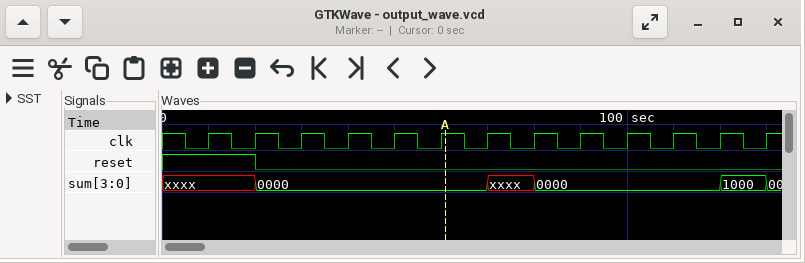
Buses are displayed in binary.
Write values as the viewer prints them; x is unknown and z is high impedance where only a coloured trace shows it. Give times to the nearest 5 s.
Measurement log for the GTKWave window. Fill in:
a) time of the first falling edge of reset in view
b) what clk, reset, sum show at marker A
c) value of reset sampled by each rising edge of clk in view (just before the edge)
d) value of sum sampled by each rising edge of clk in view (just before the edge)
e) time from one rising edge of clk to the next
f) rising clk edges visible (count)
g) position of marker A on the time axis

20 s
clk=1, reset=0, sum=0000
1 1 0 0 0 0 0 0 0 0 0 0 0
xxxx, xxxx, 0000, 0000, 0000, 0000, 0000, xxxx, 0000, 0000, 0000, 0000, 1000
10 s
13
60 s
